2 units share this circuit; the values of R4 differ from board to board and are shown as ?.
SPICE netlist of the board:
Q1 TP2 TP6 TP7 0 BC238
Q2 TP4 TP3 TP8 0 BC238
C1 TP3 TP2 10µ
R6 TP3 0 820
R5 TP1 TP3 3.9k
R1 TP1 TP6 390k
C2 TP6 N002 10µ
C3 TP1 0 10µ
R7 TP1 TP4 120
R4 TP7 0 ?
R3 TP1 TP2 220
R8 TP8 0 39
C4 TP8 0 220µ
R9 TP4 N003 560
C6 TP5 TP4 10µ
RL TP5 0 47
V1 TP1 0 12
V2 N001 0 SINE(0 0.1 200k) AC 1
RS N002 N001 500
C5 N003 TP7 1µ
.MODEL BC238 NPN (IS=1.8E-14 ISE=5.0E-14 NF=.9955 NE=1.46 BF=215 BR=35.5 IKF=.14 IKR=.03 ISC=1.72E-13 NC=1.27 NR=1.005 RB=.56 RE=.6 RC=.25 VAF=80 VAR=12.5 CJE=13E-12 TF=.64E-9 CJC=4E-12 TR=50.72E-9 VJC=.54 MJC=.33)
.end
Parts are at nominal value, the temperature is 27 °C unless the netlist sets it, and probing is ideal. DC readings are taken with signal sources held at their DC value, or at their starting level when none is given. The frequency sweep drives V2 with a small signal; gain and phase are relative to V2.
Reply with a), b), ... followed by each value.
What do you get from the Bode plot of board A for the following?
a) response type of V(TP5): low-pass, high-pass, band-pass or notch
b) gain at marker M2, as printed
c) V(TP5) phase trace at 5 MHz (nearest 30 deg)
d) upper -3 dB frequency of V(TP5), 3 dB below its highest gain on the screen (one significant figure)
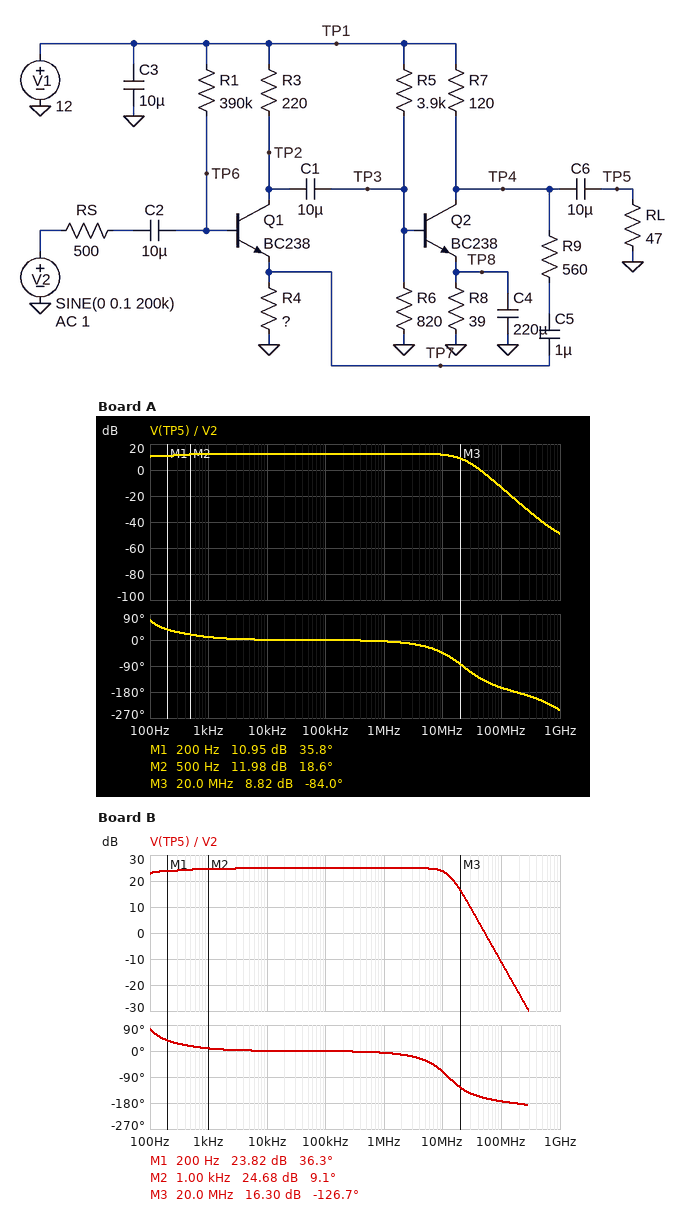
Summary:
a) low-pass
b) 11.98 dB
c) -30 deg
d) 20 MHz
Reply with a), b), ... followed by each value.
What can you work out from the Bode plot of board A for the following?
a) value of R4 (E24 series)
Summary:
a) 120 Ω
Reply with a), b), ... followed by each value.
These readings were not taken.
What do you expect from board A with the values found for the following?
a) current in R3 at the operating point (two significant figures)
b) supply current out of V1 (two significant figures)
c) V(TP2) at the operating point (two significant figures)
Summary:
a) 5.3 mA
b) 39 mA
c) 11 V
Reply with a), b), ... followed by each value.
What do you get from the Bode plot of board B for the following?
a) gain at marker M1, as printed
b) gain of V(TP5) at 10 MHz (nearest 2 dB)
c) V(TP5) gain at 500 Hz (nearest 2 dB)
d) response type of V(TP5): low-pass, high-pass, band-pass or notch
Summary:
a) 23.82 dB
b) 24 dB
c) 24 dB
d) low-pass
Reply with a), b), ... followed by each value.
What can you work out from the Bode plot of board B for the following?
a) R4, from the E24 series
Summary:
a) 24 Ω
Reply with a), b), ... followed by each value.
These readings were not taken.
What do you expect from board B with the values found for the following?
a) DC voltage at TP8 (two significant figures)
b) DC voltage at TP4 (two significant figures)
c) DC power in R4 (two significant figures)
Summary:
a) 1.2 V
b) 8.3 V
c) 760 µW
